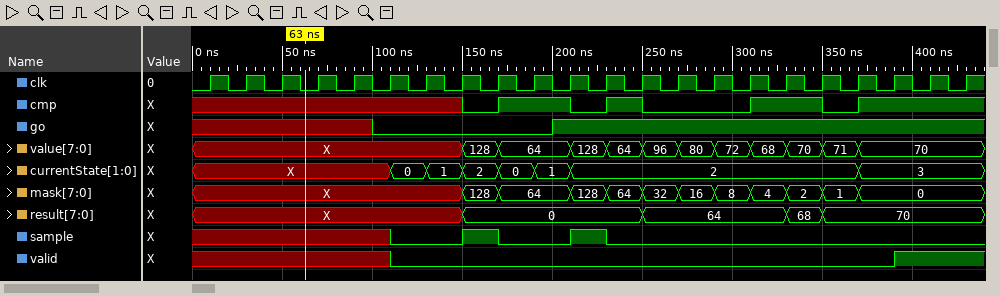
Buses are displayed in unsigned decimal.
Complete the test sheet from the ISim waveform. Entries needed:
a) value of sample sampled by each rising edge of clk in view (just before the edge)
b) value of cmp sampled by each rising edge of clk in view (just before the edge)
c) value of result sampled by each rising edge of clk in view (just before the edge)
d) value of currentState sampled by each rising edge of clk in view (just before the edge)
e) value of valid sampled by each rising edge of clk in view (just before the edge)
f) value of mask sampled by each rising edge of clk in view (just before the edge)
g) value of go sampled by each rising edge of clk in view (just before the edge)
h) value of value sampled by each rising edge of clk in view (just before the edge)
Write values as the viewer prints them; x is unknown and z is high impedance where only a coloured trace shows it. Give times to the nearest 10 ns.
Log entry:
x x x x x x 0 0 1 0 0 1 0 0 0 0 0 0 0 0 0 0
x x x x x x x x 0 1 1 0 1 0 0 0 1 1 0 1 1 1
X, X, X, X, X, X, X, X, 0, 0, 0, 0, 0, 64, 64, 64, 64, 68, 70, 70, 70, 70
X, X, X, X, X, X, 0, 1, 2, 0, 1, 2, 2, 2, 2, 2, 2, 2, 2, 3, 3, 3
x x x x x x 0 0 0 0 0 0 0 0 0 0 0 0 0 0 1 1
X, X, X, X, X, X, X, X, 128, 64, 64, 128, 64, 32, 16, 8, 4, 2, 1, 0, 0, 0
x x x x x 0 0 0 0 0 1 1 1 1 1 1 1 1 1 1 1 1
X, X, X, X, X, X, X, X, 128, 64, 64, 128, 64, 96, 80, 72, 68, 70, 71, 70, 70, 70
